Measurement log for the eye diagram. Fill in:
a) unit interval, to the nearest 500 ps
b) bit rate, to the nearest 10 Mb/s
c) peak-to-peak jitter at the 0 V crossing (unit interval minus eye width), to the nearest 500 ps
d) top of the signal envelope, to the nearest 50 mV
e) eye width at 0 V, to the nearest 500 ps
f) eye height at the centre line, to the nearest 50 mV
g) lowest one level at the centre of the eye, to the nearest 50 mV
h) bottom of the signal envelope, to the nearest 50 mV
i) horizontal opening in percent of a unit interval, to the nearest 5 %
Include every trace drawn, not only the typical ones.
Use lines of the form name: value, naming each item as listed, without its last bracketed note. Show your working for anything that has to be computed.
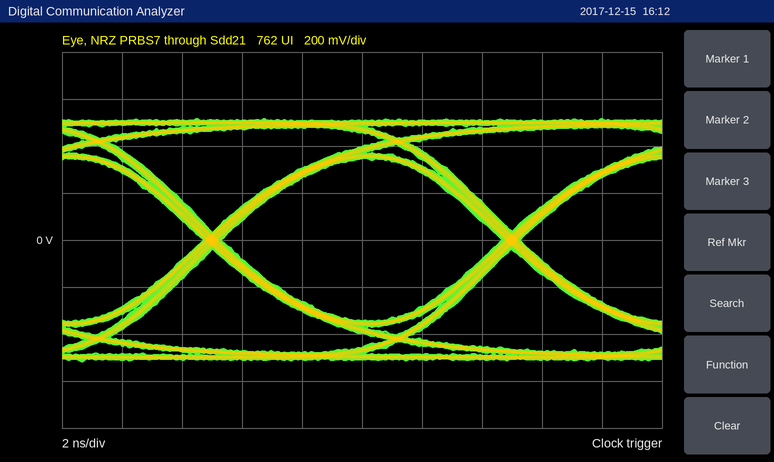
unit interval, to the nearest 500 ps: 10.0 ns
bit rate, to the nearest 10 Mb/s: 100 Mb/s
peak-to-peak jitter at the 0 V crossing (unit interval minus eye width), to the nearest 500 ps: 500 ps
top of the signal envelope, to the nearest 50 mV: 500 mV
eye width at 0 V, to the nearest 500 ps: 9.5 ns
eye height at the centre line, to the nearest 50 mV: 700 mV
lowest one level at the centre of the eye, to the nearest 50 mV: 350 mV
bottom of the signal envelope, to the nearest 50 mV: -500 mV
horizontal opening in percent of a unit interval, to the nearest 5 %: 9.5 ns / 10.0 ns ≈ 95 %
